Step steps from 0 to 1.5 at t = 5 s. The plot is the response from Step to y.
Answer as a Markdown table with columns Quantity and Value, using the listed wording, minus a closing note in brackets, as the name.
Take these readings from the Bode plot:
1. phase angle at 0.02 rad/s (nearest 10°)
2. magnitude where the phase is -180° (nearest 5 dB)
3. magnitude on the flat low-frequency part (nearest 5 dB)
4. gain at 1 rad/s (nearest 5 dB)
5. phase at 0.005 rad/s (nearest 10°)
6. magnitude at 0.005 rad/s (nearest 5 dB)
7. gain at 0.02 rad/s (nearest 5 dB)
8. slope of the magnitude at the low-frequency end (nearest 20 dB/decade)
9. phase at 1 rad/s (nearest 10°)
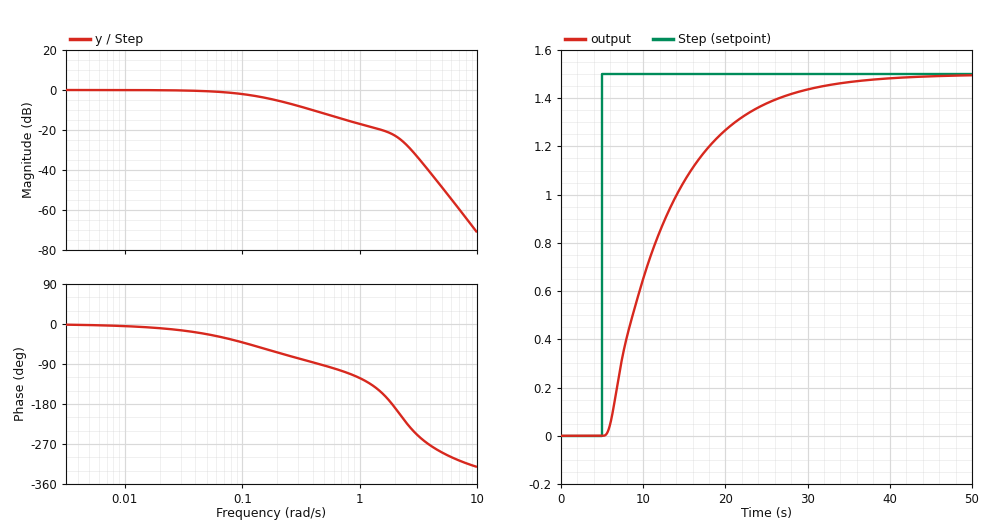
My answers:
| Quantity | Value |
|---|---|
| phase angle at 0.02 rad/s | -10° |
| magnitude where the phase is -180° | -20 dB |
| magnitude on the flat low-frequency part | 0 dB |
| gain at 1 rad/s | -15 dB |
| phase at 0.005 rad/s | 0° |
| magnitude at 0.005 rad/s | 0 dB |
| gain at 0.02 rad/s | 0 dB |
| slope of the magnitude at the low-frequency end | 0 dB/decade |
| phase at 1 rad/s | -120° |
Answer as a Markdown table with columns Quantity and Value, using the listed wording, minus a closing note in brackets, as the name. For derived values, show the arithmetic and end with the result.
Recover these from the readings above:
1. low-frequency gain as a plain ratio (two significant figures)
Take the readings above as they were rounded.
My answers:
| Quantity | Value |
|---|---|
| low-frequency gain as a plain ratio | 10^(0 / 20) = 1.0 |
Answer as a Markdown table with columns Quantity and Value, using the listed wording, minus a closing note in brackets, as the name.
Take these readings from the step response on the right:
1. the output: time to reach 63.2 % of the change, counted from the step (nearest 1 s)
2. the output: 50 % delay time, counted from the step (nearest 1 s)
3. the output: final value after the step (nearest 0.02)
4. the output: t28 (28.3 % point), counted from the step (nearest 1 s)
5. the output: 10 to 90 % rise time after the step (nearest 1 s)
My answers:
| Quantity | Value |
|---|---|
| the output: time to reach 63.2 % of the change, counted from the step | 8 s |
| the output: 50 % delay time, counted from the step | 6 s |
| the output: final value after the step | 1.50 |
| the output: t28 (28.3 % point), counted from the step | 3 s |
| the output: 10 to 90 % rise time after the step | 17 s |
